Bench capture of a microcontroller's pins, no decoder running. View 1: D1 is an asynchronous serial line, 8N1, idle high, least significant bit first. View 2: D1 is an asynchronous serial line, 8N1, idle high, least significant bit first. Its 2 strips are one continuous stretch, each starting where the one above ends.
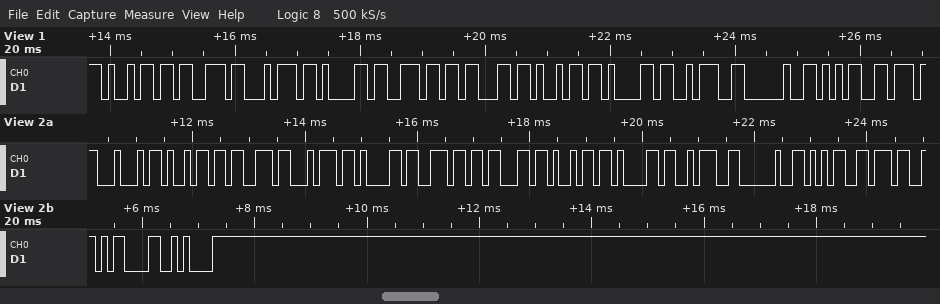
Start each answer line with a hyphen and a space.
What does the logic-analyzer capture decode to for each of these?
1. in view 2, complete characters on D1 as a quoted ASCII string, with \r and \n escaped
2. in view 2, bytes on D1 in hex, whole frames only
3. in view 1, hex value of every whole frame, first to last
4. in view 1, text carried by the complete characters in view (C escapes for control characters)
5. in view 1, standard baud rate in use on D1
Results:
- "Distancia: 57\r\n"
- 44 69 73 74 61 6E 63 69 61 3A 20 35 37 0D 0A
- 69 73 74 61 6E 63 69 61 3A 20 35
- "istancia: 5"
- 9600 baud
